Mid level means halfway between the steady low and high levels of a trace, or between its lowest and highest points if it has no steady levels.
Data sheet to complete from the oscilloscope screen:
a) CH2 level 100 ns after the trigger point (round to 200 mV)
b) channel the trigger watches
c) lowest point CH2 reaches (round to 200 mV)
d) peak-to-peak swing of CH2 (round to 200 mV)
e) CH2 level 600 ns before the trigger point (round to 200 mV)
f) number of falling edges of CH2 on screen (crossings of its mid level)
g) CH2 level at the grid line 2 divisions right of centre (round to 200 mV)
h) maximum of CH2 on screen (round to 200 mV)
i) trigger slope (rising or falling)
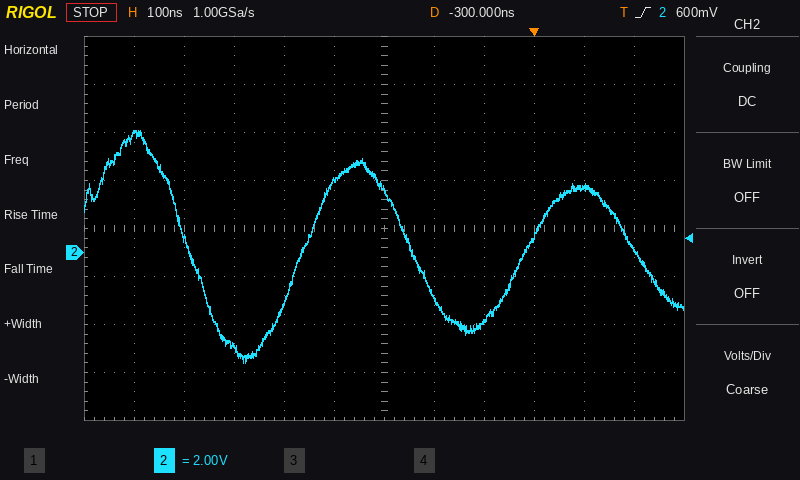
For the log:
2.8 V
CH2
-4.6 V
9.6 V
-4.0 V
3
-2.8 V
5.0 V
rising
